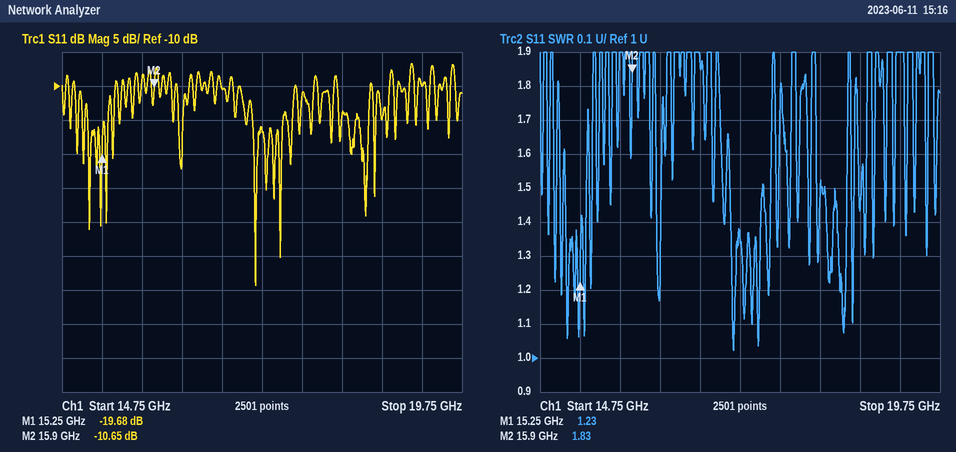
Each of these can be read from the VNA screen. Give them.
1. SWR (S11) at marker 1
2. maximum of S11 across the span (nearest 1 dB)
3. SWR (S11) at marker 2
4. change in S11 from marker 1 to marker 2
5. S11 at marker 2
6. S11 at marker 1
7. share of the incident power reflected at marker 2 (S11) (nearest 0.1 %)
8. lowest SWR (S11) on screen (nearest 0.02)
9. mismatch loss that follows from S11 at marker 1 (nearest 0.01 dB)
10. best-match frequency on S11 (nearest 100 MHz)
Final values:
1.23
-7 dB
1.83
9.03 dB
-10.65 dB
-19.68 dB
8.6 %
1.02
0.05 dB
17.2 GHz
